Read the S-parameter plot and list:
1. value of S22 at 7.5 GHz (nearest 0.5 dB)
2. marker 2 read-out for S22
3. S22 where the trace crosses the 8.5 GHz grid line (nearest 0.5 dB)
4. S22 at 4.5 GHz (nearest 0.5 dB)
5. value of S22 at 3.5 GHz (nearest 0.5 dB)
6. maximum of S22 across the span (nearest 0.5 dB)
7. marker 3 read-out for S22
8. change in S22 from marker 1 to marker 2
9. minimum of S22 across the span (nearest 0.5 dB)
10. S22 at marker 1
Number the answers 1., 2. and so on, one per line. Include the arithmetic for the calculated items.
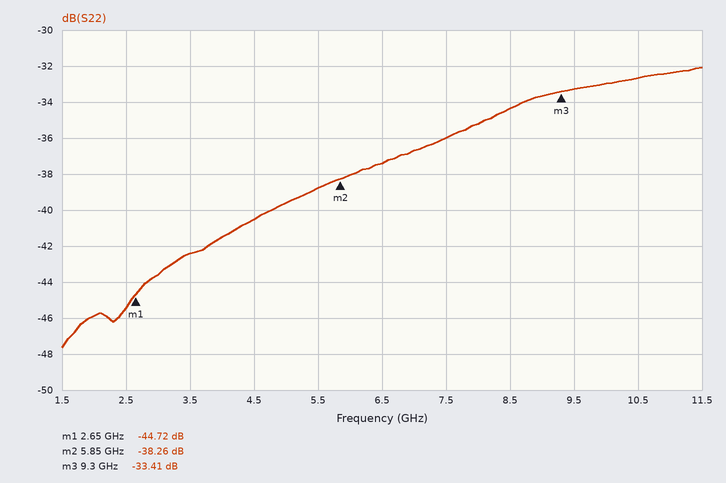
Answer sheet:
1. -36.0 dB
2. -38.26 dB
3. -34.5 dB
4. -40.5 dB
5. -42.5 dB
6. -32.0 dB
7. -33.41 dB
8. -38.26 − (-44.72) = 6.46 dB
9. -47.5 dB
10. -44.72 dB
